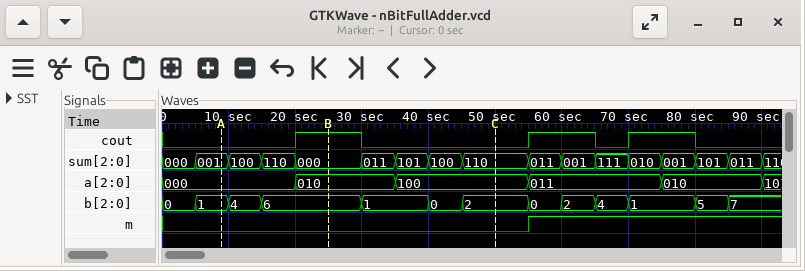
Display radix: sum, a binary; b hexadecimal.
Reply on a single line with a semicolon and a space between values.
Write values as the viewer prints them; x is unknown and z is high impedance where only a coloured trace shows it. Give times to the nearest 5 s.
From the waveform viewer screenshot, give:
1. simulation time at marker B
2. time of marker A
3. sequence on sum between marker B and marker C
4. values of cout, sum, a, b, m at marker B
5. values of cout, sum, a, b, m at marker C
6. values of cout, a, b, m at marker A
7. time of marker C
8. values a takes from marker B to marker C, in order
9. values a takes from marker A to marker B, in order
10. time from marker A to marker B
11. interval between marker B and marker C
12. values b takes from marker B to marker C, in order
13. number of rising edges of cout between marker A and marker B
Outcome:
25 s; 10 s; 000, 011, 101, 100, 110; cout=1, sum=000, a=010, b=6, m=0; cout=0, sum=110, a=100, b=2, m=0; cout=0, a=000, b=1, m=0; 50 s; 010, 100; 000, 010; 15 s; 25 s; 6, 1, 0, 2; 1
